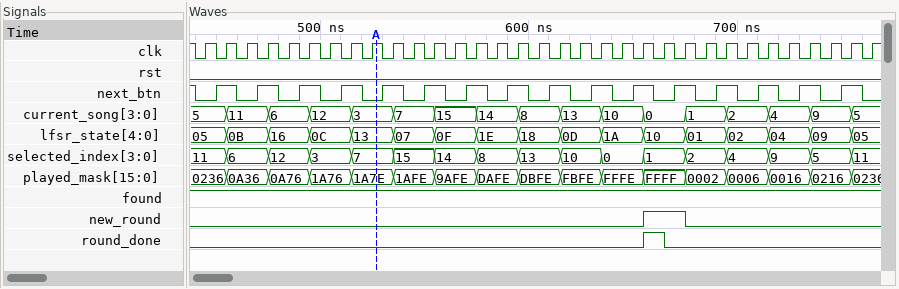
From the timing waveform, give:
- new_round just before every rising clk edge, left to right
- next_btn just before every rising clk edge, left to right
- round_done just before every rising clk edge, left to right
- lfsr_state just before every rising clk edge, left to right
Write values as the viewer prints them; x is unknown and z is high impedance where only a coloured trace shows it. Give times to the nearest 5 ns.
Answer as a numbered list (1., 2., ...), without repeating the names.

1. 0 0 0 0 0 0 0 0 0 0 0 0 0 0 0 0 0 0 0 0 0 0 1 1 0 0 0 0 0 0 0 0 0
2. 0 1 0 1 0 1 0 1 0 1 0 1 0 1 0 1 0 1 0 1 0 1 0 1 0 1 0 1 0 1 0 1 0
3. 0 0 0 0 0 0 0 0 0 0 0 0 0 0 0 0 0 0 0 0 0 0 1 0 0 0 0 0 0 0 0 0 0
4. 05, 05, 0B, 0B, 16, 16, 0C, 0C, 13, 13, 07, 07, 0F, 0F, 1E, 1E, 18, 18, 0D, 0D, 1A, 1A, 10, 10, 01, 01, 02, 02, 04, 04, 09, 09, 05
